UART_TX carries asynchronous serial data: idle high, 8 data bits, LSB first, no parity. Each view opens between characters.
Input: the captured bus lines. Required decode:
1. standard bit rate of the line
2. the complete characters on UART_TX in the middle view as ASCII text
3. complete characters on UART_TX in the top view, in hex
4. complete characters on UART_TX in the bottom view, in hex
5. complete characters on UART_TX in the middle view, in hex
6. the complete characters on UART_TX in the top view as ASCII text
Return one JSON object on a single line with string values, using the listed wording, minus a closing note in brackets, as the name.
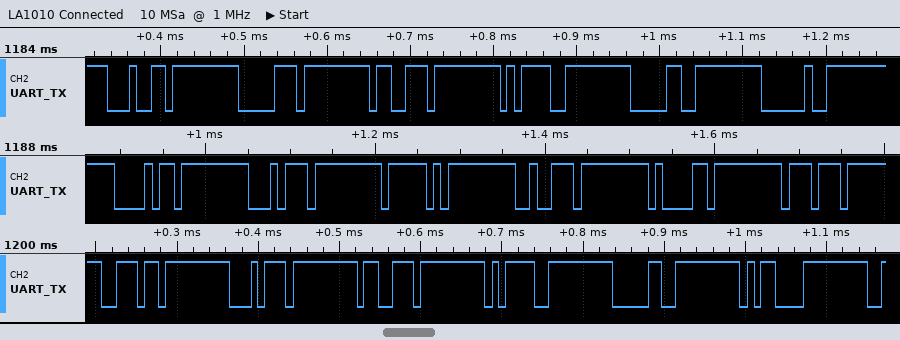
{"standard bit rate of the line": "115200 baud", "the complete characters on UART_TX in the middle view as ASCII text": "\"ht_raw\"", "complete characters on UART_TX in the top view, in hex": "64, 70, 73, 3D, 30, 20", "complete characters on UART_TX in the bottom view, in hex": "6E, 74, 73, 3D, 30, 0D", "complete characters on UART_TX in the middle view, in hex": "68, 74, 5F, 72, 61, 77", "the complete characters on UART_TX in the top view as ASCII text": "\"dps=0 \""}
